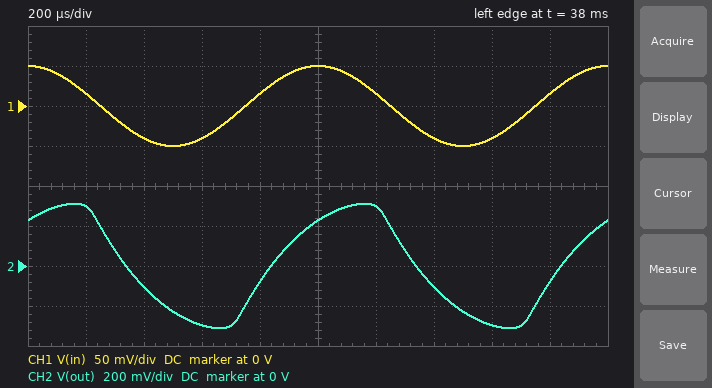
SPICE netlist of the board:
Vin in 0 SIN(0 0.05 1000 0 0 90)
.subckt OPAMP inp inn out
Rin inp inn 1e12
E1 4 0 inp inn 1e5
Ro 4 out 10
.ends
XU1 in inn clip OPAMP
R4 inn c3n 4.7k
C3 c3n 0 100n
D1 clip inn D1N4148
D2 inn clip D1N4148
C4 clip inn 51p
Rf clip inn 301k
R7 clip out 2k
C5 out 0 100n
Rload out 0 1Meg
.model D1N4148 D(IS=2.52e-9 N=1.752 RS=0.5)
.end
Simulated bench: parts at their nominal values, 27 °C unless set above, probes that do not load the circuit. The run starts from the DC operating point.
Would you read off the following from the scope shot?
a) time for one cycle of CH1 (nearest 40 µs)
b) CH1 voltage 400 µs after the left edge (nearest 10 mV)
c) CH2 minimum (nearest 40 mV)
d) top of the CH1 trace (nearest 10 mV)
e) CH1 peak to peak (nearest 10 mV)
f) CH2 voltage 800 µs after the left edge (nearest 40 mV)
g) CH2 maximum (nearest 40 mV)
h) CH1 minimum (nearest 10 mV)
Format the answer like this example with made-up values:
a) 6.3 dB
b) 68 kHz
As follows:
a) 1.00 ms
b) -40 mV
c) -320 mV
d) 50 mV
e) 100 mV
f) -80 mV
g) 320 mV
h) -50 mV
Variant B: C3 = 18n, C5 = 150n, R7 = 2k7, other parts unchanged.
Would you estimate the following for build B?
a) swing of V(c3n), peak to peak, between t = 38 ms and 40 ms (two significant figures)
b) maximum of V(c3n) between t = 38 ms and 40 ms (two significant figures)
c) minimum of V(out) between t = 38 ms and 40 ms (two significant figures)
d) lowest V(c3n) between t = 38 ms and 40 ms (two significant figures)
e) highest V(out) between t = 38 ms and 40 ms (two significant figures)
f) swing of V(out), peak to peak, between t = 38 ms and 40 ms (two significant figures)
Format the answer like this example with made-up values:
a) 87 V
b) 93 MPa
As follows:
a) 88 mV
b) 44 mV
c) -170 mV
d) -44 mV
e) 170 mV
f) 340 mV
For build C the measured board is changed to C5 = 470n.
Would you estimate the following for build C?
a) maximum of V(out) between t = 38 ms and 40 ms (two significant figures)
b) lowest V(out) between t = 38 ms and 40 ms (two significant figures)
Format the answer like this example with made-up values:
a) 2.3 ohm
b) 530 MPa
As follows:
a) 93 mV
b) -93 mV
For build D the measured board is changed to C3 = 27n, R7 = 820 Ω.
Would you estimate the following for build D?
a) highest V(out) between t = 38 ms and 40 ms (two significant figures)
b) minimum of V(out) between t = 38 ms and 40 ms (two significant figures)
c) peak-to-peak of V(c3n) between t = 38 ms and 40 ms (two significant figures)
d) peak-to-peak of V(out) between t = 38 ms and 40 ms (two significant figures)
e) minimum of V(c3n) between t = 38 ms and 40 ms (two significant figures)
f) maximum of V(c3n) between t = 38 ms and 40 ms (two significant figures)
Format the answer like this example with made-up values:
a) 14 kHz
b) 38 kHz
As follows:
a) 370 mV
b) -370 mV
c) 78 mV
d) 740 mV
e) -39 mV
f) 39 mV
